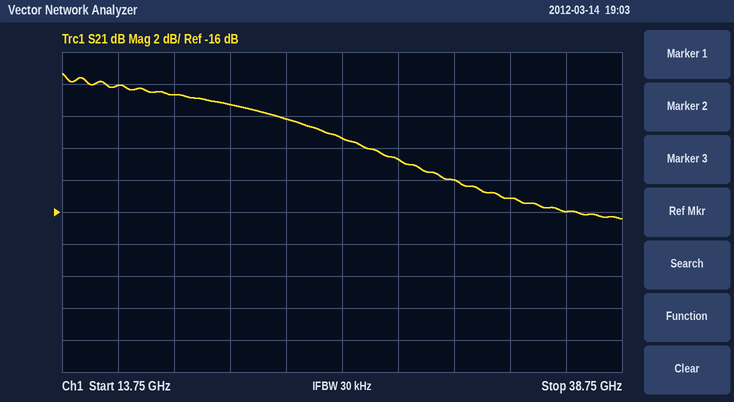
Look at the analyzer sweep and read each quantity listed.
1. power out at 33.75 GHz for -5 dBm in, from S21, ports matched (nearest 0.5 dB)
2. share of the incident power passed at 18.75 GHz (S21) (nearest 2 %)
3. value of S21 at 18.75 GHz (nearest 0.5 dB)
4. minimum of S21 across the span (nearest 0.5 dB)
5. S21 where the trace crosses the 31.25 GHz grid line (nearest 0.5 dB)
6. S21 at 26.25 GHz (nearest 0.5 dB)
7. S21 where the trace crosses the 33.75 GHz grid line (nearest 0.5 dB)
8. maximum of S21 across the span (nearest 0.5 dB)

-20.0 dBm
14 %
-8.5 dB
-16.5 dB
-14.0 dB
-11.5 dB
-15.0 dB
-7.5 dB
